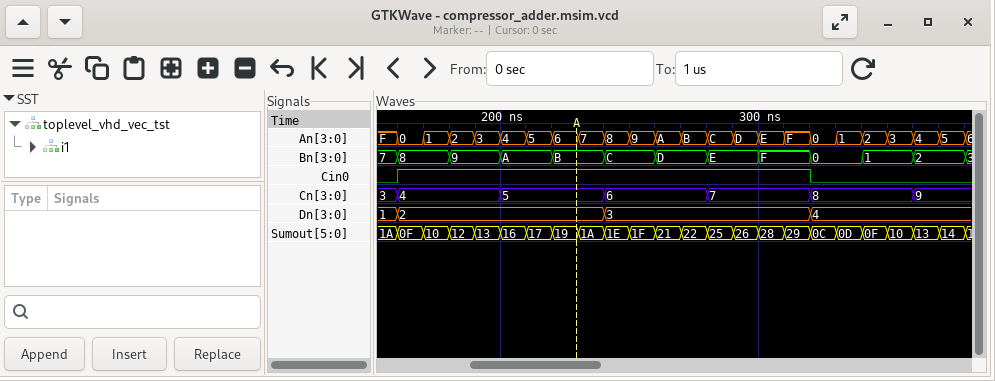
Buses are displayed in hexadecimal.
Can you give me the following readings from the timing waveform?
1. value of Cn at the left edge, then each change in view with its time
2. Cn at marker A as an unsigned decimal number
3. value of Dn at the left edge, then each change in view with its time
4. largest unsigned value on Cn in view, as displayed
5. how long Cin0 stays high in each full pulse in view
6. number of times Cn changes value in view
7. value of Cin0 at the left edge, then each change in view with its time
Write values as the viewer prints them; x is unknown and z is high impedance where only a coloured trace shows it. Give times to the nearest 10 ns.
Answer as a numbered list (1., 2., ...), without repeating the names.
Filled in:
1. 3, 4 at 160 ns, 5 at 200 ns, 6 at 240 ns, 7 at 280 ns, 8 at 320 ns, 9 at 360 ns
2. 5
3. 1, 2 at 160 ns, 3 at 240 ns, 4 at 320 ns
4. 9
5. 160 ns
6. 6
7. 0, 1 at 160 ns, 0 at 320 ns
